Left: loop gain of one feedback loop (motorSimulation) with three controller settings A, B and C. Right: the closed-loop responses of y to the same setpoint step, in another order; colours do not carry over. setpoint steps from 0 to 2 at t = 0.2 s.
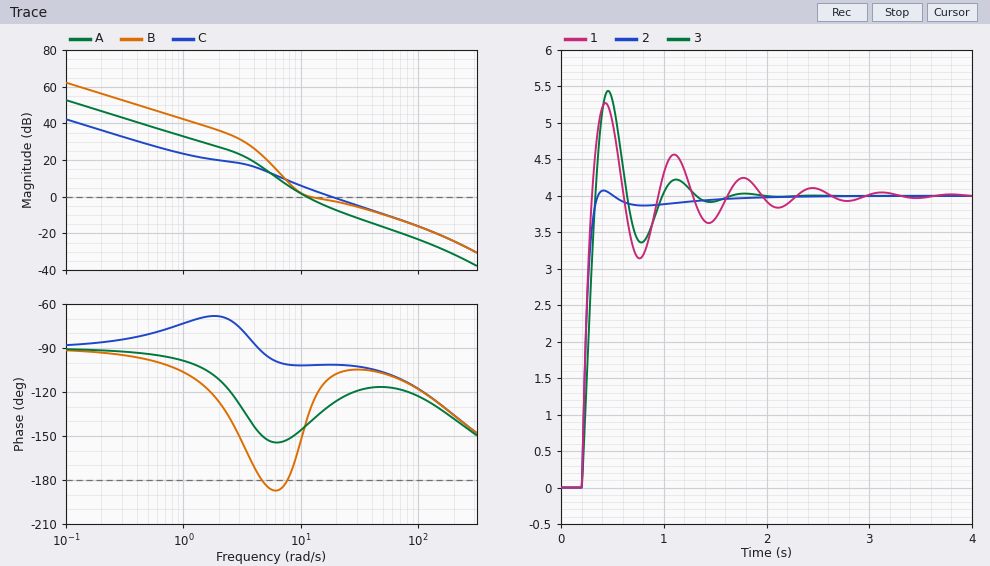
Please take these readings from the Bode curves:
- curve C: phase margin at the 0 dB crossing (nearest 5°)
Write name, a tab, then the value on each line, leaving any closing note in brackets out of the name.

curve C: phase margin at the 0 dB crossing	80°
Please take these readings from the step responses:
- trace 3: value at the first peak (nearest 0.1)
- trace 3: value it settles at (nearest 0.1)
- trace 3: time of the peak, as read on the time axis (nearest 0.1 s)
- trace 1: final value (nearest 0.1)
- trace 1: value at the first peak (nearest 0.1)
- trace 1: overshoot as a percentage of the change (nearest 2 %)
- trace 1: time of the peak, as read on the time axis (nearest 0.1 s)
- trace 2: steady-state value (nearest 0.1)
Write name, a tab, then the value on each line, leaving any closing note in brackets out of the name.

trace 3: value at the first peak	5.4
trace 3: value it settles at	4.0
trace 3: time of the peak, as read on the time axis	0.5 s
trace 1: final value	4.0
trace 1: value at the first peak	5.3
trace 1: overshoot as a percentage of the change	32 %
trace 1: time of the peak, as read on the time axis	0.4 s
trace 2: steady-state value	4.0
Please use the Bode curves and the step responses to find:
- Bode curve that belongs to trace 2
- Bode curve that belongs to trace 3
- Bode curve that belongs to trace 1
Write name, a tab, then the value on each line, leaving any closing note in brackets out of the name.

Bode curve that belongs to trace 2	C
Bode curve that belongs to trace 3	A
Bode curve that belongs to trace 1	B
